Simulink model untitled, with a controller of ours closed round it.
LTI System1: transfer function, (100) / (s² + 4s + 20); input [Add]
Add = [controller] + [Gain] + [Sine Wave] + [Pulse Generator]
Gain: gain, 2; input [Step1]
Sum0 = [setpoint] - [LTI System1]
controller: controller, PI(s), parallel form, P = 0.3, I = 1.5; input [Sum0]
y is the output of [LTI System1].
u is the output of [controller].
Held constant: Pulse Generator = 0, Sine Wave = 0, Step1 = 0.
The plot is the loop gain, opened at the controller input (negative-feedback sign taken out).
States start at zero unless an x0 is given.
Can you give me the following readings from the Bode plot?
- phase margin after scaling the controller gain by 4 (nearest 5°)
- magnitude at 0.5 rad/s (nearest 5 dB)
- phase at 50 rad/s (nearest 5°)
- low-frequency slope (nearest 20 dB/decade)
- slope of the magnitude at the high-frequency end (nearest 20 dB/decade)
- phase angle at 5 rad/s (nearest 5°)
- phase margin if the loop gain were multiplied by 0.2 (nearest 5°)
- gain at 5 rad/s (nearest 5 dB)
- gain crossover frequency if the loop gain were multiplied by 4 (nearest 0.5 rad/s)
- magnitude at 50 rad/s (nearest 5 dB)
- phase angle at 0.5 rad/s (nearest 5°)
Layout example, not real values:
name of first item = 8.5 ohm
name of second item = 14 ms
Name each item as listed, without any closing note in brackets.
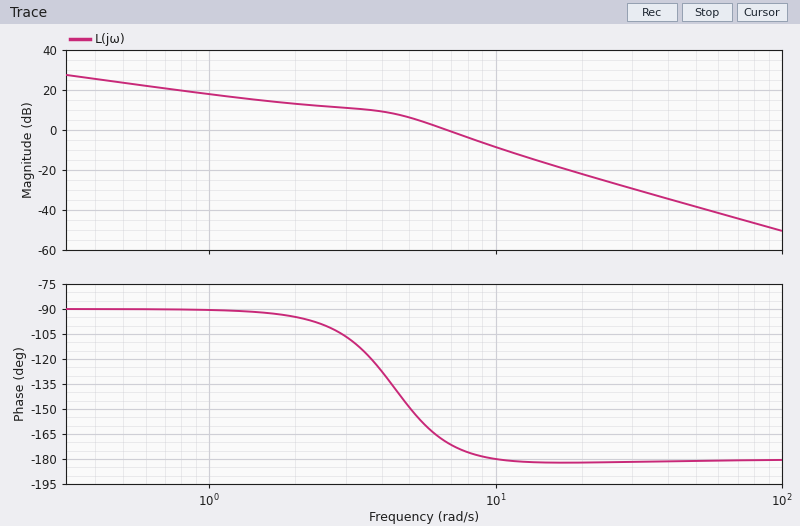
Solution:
phase margin after scaling the controller gain by 4 = 0°
magnitude at 0.5 rad/s = 25 dB
phase at 50 rad/s = -180°
low-frequency slope = -20 dB/decade
slope of the magnitude at the high-frequency end = -40 dB/decade
phase angle at 5 rad/s = -150°
phase margin if the loop gain were multiplied by 0.2 = 85°
gain at 5 rad/s = 5 dB
gain crossover frequency if the loop gain were multiplied by 4 = 12.0 rad/s
magnitude at 50 rad/s = -40 dB
phase angle at 0.5 rad/s = -90°
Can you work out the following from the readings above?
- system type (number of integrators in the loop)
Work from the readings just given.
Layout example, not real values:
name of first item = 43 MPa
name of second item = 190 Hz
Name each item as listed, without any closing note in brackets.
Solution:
system type = 1
